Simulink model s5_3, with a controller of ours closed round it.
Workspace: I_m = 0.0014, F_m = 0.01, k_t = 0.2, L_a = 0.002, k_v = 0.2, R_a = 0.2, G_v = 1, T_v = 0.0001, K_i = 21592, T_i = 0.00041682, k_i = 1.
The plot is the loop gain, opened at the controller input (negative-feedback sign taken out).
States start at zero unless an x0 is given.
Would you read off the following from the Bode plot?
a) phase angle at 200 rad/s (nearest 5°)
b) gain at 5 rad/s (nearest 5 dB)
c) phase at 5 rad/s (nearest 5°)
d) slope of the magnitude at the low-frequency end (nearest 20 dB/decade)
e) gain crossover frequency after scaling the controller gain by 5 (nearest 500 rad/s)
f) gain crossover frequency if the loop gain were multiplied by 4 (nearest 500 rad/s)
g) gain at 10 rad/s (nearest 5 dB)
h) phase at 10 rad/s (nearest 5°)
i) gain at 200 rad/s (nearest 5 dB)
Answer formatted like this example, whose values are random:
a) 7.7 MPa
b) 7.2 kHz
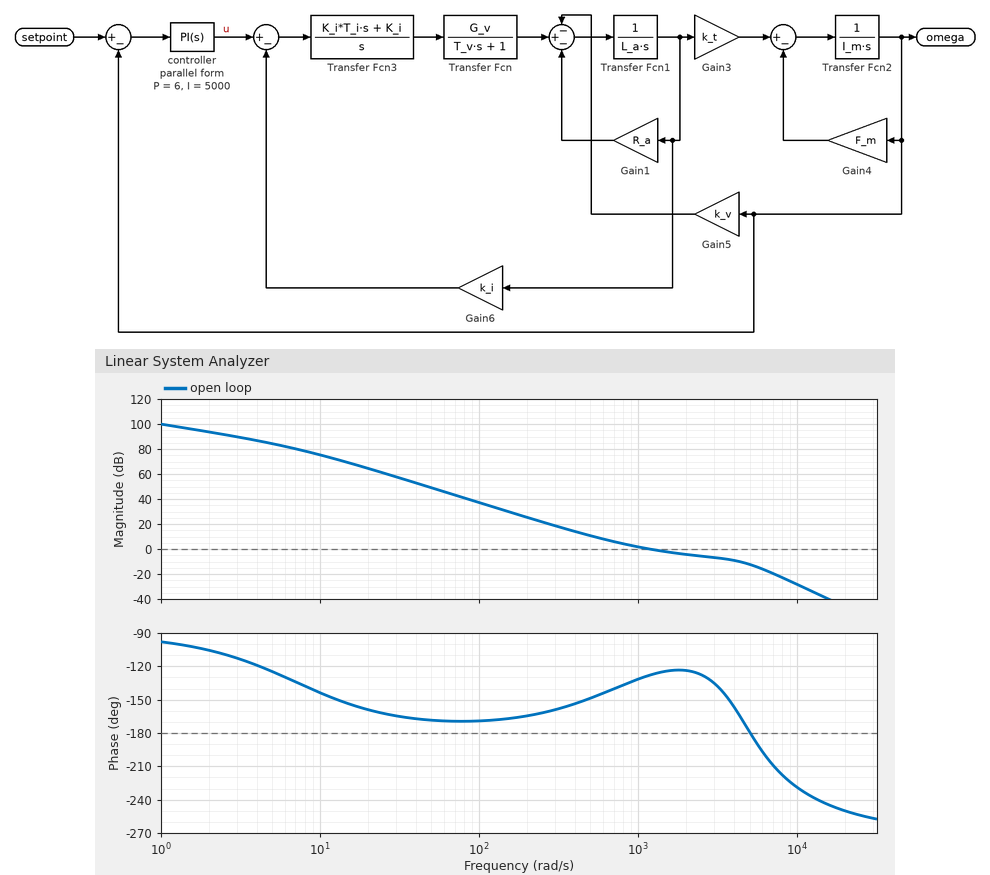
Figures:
a) -165°
b) 85 dB
c) -125°
d) -20 dB/decade
e) 5500 rad/s
f) 5000 rad/s
g) 75 dB
h) -145°
i) 25 dB
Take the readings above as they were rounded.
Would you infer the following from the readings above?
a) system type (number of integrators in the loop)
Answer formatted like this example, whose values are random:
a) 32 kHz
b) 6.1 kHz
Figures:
a) 1
